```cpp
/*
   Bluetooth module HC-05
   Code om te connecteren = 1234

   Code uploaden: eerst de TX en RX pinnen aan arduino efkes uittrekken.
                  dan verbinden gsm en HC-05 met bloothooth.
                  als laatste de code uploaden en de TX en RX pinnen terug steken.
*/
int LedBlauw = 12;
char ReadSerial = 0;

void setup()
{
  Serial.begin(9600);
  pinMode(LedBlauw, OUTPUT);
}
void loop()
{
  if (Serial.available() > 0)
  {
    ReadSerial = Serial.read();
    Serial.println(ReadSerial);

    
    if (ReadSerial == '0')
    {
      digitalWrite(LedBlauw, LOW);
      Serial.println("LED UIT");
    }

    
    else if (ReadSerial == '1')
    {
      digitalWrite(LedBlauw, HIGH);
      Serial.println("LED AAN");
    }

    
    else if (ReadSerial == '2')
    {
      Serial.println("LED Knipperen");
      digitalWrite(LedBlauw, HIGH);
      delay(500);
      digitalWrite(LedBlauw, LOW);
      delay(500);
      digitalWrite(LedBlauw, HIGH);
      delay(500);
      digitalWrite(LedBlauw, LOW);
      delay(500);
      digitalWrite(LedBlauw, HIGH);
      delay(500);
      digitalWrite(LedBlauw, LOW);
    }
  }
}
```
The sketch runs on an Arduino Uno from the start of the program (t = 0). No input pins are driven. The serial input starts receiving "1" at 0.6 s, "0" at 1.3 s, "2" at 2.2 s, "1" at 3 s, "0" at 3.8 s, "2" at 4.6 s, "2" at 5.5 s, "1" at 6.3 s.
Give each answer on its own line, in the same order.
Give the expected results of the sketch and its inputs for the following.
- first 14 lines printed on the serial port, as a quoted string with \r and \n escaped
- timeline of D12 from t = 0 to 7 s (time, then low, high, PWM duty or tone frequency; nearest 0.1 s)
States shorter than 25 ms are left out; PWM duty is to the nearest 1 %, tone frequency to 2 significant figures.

"1\r\nLED AAN\r\n0\r\nLED UIT\r\n2\r\nLED Knipperen\r\n1\r\nLED AAN\r\n0\r\nLED UIT\r\n2\r\nLED Knipperen\r\n2\r\nLED Knipperen\r\n"
0 s low; 0.6 s high; 1.3 s low; 2.2 s high; 2.7 s low; 3.2 s high; 3.7 s low; 4.2 s high; 5.2 s low; 5.7 s high; 6.2 s low; 6.7 s high
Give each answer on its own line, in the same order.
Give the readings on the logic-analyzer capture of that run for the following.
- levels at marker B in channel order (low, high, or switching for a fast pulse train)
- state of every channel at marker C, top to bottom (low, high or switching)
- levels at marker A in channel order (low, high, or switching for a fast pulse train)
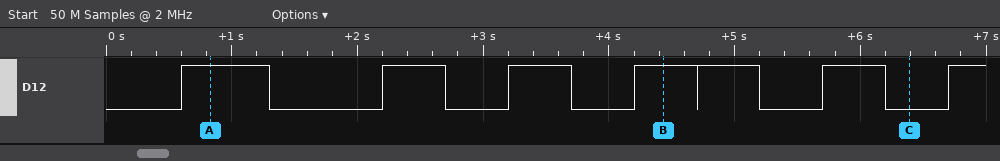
D12 high
D12 low
D12 high
